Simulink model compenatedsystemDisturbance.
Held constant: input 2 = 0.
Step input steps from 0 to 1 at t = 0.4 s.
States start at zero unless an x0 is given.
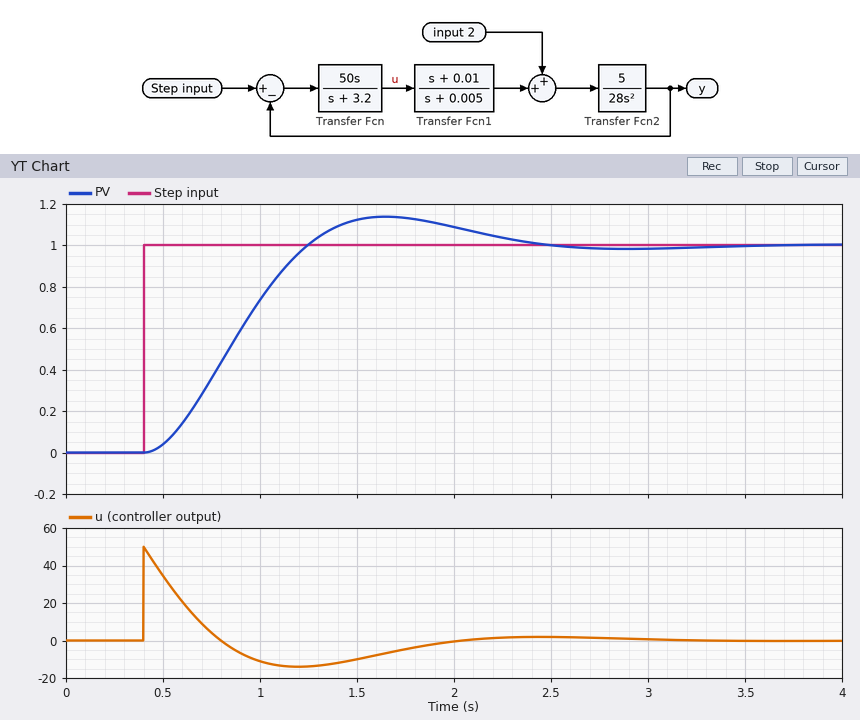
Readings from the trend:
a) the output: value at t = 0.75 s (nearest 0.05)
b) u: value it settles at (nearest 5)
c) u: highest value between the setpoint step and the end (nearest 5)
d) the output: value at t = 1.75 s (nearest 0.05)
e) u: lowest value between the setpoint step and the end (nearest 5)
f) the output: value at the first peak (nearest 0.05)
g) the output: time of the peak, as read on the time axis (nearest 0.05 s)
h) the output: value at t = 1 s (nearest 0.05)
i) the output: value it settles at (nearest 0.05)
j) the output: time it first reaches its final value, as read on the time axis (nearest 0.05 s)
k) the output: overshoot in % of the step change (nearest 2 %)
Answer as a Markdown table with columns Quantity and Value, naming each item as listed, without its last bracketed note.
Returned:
| Quantity | Value |
|---|---|
| the output: value at t = 0.75 s | 0.35 |
| u: value it settles at | 0 |
| u: highest value between the setpoint step and the end | 50 |
| the output: value at t = 1.75 s | 1.15 |
| u: lowest value between the setpoint step and the end | -15 |
| the output: value at the first peak | 1.15 |
| the output: time of the peak, as read on the time axis | 1.65 s |
| the output: value at t = 1 s | 0.75 |
| the output: value it settles at | 1.00 |
| the output: time it first reaches its final value, as read on the time axis | 1.25 s |
| the output: overshoot in % of the step change | 14 % |
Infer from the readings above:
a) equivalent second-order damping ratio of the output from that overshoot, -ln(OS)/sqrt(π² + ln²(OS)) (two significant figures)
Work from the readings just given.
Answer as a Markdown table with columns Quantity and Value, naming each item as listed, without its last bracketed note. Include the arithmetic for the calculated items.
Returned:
| Quantity | Value |
|---|---|
| equivalent second-order damping ratio of the output from that overshoot, -ln(OS)/sqrt(π² + ln²(OS)) | ln(0.14) = -1.966; 1.966 / sqrt(9.870 + 3.866) = 0.53 |
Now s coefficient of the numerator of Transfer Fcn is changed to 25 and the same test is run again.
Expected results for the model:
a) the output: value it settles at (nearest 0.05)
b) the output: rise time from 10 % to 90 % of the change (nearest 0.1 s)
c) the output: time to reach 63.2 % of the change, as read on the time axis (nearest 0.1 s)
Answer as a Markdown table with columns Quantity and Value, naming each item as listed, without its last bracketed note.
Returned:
| Quantity | Value |
|---|---|
| the output: value it settles at | 1.00 |
| the output: rise time from 10 % to 90 % of the change | 1.1 s |
| the output: time to reach 63.2 % of the change, as read on the time axis | 1.3 s |
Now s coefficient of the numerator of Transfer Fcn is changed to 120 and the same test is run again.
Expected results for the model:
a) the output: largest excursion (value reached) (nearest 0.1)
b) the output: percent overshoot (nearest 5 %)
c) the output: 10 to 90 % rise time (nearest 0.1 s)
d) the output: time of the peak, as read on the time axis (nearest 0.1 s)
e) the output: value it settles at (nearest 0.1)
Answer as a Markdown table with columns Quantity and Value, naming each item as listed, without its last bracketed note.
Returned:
| Quantity | Value |
|---|---|
| the output: largest excursion (value reached) | 1.3 |
| the output: percent overshoot | 30 % |
| the output: 10 to 90 % rise time | 0.3 s |
| the output: time of the peak, as read on the time axis | 1.1 s |
| the output: value it settles at | 1.0 |
